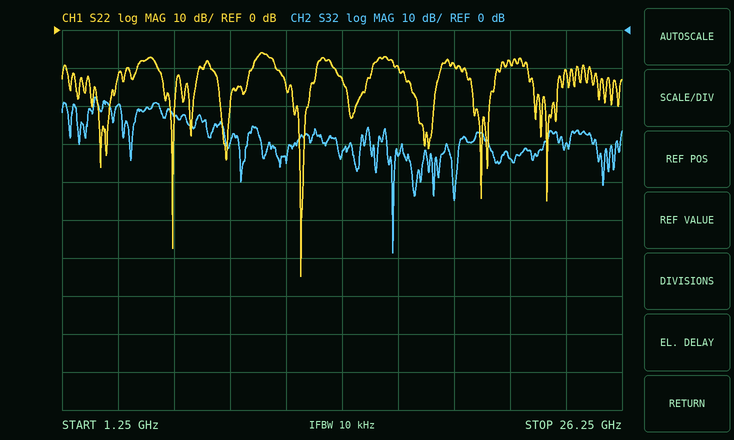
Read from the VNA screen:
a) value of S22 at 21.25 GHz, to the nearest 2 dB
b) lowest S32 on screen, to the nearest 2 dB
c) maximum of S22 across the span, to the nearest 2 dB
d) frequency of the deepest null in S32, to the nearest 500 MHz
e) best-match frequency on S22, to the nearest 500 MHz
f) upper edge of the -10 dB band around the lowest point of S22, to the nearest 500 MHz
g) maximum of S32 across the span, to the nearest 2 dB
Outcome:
-8 dB
-58 dB
-6 dB
16.0 GHz
12.0 GHz
12.5 GHz
-18 dB
